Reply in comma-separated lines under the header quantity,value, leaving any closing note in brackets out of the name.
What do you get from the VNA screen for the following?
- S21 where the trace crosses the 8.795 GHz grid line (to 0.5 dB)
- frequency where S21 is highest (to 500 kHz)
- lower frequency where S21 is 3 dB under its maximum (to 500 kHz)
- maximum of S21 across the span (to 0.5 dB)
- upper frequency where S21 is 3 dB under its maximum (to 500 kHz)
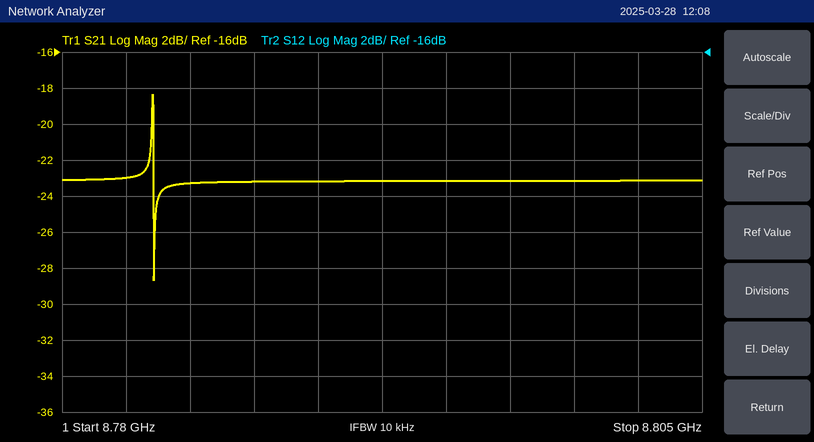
quantity,value
S21 where the trace crosses the 8.795 GHz grid line,-23.0 dB
frequency where S21 is highest,8.7835 GHz
lower frequency where S21 is 3 dB under its maximum,8.7835 GHz
maximum of S21 across the span,-18.5 dB
upper frequency where S21 is 3 dB under its maximum,8.7835 GHz
